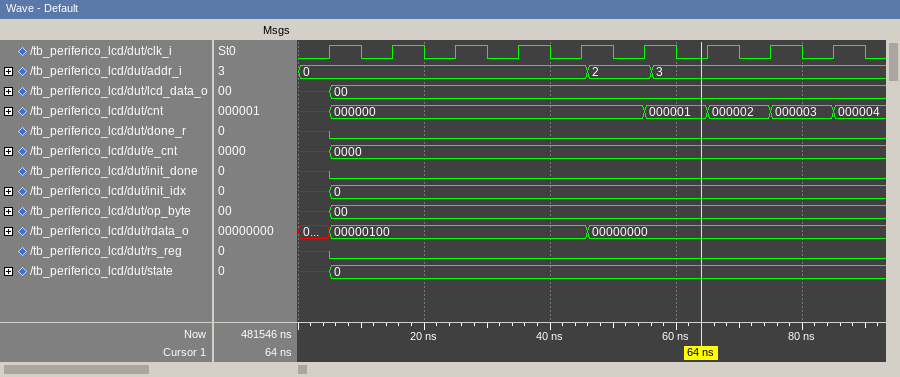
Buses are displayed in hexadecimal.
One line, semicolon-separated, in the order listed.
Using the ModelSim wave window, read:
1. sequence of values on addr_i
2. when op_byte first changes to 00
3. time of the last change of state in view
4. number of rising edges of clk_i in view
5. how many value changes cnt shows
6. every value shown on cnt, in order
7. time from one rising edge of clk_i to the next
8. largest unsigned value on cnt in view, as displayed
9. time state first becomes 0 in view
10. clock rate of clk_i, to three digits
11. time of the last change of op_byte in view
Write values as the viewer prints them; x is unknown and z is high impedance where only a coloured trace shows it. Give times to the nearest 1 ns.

0, 2, 3; 5 ns; 5 ns; 9; 5; x, 000000, 000001, 000002, 000003, 000004; 10 ns; 000004; 5 ns; 100 MHz; 5 ns
